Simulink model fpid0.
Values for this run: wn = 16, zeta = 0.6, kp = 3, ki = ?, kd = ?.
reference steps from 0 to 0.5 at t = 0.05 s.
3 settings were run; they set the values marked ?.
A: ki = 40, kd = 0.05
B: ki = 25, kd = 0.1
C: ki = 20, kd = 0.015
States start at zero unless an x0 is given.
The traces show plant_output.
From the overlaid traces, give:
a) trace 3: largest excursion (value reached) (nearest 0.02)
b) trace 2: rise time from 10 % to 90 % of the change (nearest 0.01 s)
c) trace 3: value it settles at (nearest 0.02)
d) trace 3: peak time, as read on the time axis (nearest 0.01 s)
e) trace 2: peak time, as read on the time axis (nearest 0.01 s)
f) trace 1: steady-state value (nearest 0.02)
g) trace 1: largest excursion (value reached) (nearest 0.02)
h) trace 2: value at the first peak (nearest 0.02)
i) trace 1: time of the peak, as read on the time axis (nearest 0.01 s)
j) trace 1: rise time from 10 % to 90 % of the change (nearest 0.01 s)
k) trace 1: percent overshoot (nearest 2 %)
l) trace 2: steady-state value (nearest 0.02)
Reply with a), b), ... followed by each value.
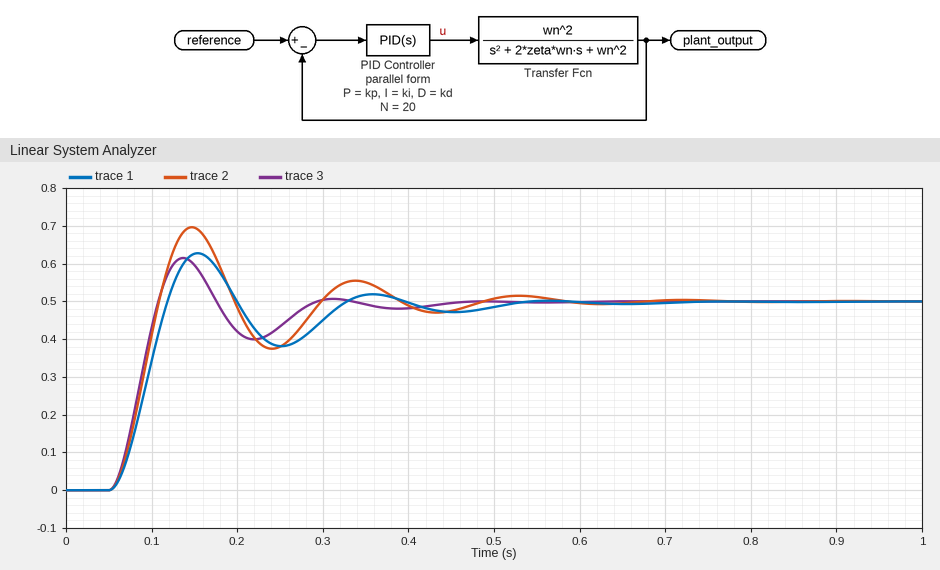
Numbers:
a) 0.62
b) 0.04 s
c) 0.50
d) 0.14 s
e) 0.15 s
f) 0.50
g) 0.62
h) 0.70
i) 0.15 s
j) 0.05 s
k) 26 %
l) 0.50
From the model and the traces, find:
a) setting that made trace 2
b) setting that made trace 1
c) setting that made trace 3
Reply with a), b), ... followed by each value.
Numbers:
a) A
b) C
c) B
